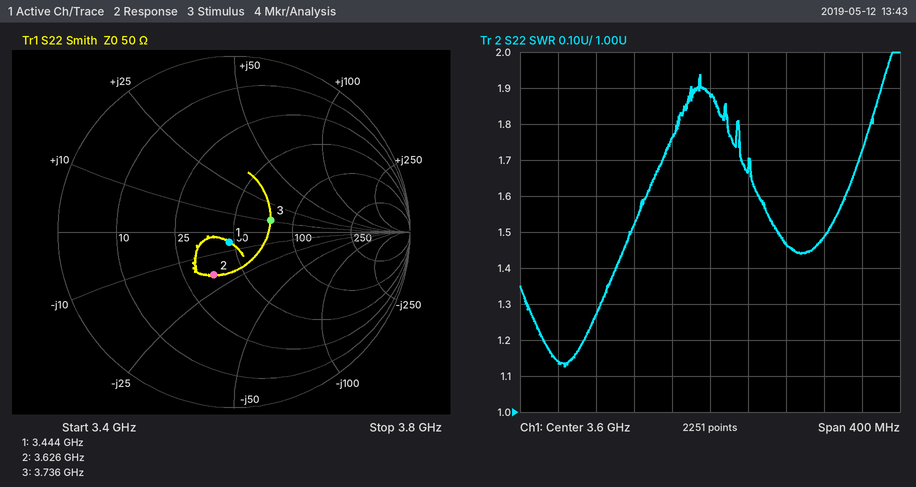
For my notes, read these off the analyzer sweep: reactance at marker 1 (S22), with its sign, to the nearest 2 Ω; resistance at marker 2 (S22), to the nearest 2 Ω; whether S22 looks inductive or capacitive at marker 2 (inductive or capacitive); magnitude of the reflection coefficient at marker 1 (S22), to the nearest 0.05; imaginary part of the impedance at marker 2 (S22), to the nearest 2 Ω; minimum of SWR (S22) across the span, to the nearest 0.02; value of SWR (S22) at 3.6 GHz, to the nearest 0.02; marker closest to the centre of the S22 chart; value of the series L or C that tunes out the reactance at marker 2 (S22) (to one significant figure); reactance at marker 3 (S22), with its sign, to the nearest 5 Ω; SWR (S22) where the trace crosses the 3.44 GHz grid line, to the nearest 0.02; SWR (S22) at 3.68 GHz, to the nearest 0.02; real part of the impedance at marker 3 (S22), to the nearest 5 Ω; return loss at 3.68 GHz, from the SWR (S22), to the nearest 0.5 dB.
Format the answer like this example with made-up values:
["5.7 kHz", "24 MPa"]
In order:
["-6 Ω", "36 Ω", "capacitive", "0.05", "-18 Ω", "1.12", "1.88", "marker 1", "800 pH", "+10 Ω", "1.14", "1.46", "75 Ω", "14.5 dB"]
